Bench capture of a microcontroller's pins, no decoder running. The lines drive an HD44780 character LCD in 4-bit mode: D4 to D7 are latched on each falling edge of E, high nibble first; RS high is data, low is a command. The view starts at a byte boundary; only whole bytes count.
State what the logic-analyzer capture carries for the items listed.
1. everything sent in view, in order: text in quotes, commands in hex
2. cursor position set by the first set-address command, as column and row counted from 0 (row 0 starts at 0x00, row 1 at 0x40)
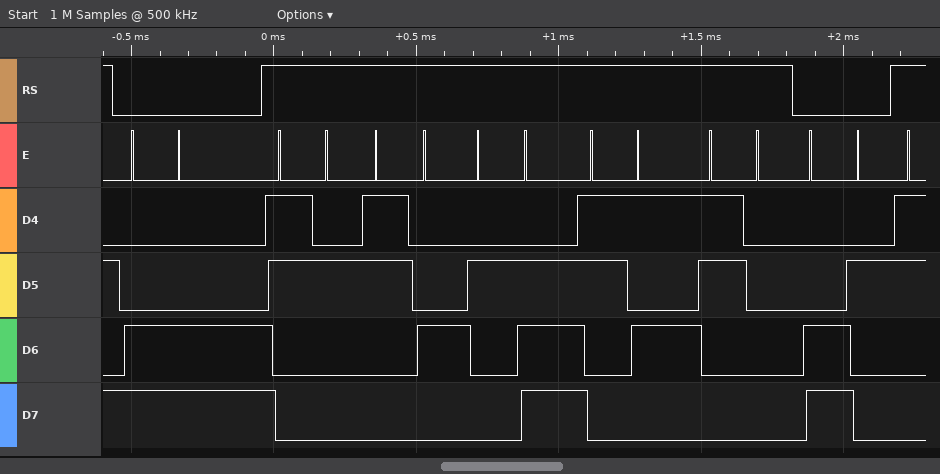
0xCC "24.50" 0xC2
column 12, row 1
